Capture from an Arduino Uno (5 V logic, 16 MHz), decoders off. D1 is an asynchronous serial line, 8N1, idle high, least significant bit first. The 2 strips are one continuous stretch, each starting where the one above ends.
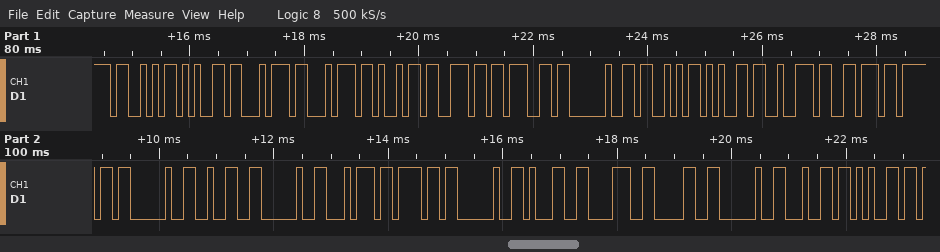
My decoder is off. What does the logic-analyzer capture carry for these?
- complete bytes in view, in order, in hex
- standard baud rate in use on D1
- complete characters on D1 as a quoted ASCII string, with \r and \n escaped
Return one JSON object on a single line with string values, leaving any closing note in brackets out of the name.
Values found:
{"complete bytes in view, in order, in hex": "53 65 74 74 69 6E 67 20 53 65 72 76 6F 20 32 20 74 6F 20 31 38 30 20 64 65", "standard baud rate in use on D1": "9600 baud", "complete characters on D1 as a quoted ASCII string, with \\r and \\n escaped": "\"Setting Servo 2 to 180 de\""}
